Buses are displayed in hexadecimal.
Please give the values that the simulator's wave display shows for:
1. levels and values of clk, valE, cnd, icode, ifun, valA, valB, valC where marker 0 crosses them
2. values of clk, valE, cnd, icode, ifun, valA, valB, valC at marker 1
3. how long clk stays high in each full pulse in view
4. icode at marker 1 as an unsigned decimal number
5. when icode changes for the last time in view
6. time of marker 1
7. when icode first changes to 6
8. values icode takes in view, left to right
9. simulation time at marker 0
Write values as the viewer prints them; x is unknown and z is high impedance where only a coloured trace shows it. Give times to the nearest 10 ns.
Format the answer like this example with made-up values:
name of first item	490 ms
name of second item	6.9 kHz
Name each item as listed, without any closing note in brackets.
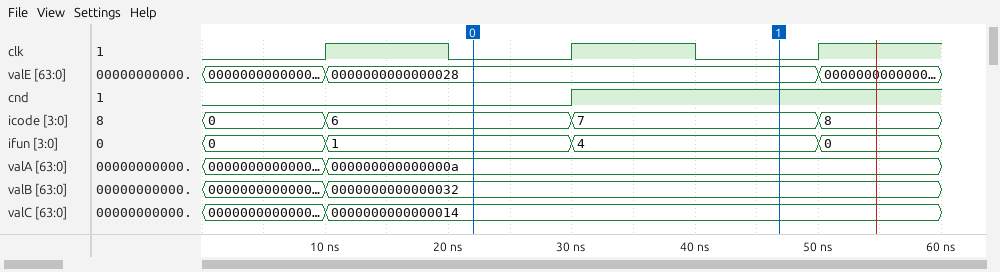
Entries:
levels and values of clk, valE, cnd, icode, ifun, valA, valB, valC where marker 0 crosses them	clk=0, valE=0000000000000028, cnd=0, icode=6, ifun=1, valA=000000000000000a, valB=0000000000000032, valC=0000000000000014
values of clk, valE, cnd, icode, ifun, valA, valB, valC at marker 1	clk=0, valE=0000000000000028, cnd=1, icode=7, ifun=4, valA=000000000000000a, valB=0000000000000032, valC=0000000000000014
how long clk stays high in each full pulse in view	10 ns, 10 ns
icode at marker 1 as an unsigned decimal number	7
when icode changes for the last time in view	50 ns
time of marker 1	50 ns
when icode first changes to 6	10 ns
values icode takes in view, left to right	0, 6, 7, 8
simulation time at marker 0	20 ns
